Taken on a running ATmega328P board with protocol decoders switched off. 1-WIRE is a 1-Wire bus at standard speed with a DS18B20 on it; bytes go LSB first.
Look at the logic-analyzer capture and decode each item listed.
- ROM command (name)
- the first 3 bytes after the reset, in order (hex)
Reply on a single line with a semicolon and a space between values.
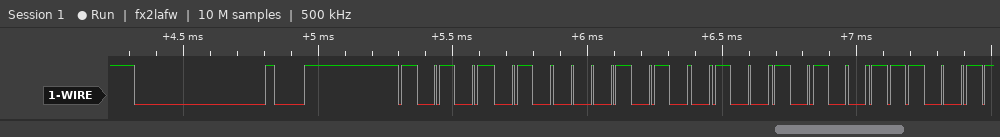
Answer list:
Match ROM; 55 28 29
